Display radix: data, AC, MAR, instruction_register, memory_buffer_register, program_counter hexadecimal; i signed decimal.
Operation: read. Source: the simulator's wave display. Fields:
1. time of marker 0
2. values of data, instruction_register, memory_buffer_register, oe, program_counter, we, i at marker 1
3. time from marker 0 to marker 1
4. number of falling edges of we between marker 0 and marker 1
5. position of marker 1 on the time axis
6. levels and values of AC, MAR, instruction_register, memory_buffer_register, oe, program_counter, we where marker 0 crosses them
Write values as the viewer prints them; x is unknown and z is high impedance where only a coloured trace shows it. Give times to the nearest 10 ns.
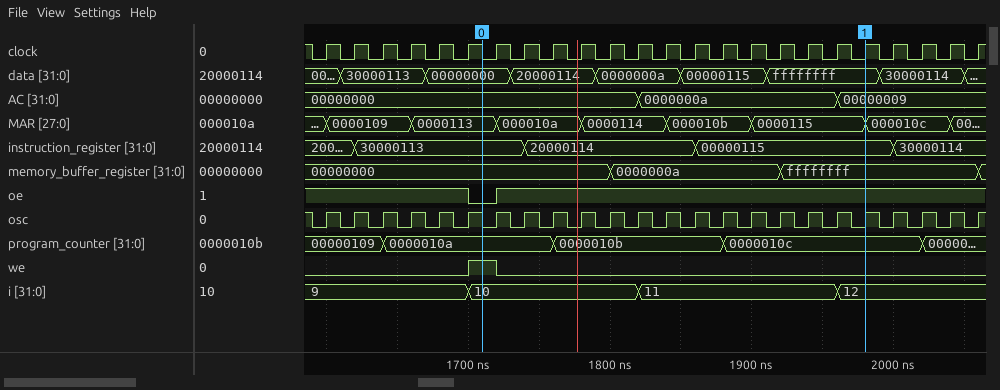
1710 ns
data=ffffffff, instruction_register=00000115, memory_buffer_register=ffffffff, oe=1, program_counter=0000010c, we=0, i=12
270 ns
1
1980 ns
AC=00000000, MAR=0000113, instruction_register=30000113, memory_buffer_register=00000000, oe=0, program_counter=0000010a, we=1
